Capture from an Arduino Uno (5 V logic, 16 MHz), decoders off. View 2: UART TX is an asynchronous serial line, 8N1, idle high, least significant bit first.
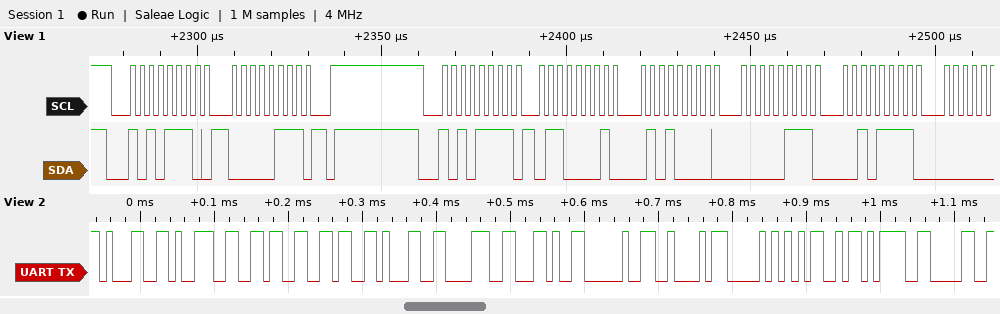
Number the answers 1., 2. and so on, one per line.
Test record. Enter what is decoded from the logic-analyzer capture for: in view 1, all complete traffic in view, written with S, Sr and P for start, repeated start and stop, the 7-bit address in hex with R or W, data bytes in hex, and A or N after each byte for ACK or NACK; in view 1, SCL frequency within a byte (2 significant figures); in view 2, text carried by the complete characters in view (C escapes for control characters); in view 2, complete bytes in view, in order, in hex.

1. S 57W A 07 A P S 57R A 61 A 50 A 07 A 2F A
2. 400 kHz
3. "196618, BPM=0"
4. 31 39 36 36 31 38 2C 20 42 50 4D 3D 30
